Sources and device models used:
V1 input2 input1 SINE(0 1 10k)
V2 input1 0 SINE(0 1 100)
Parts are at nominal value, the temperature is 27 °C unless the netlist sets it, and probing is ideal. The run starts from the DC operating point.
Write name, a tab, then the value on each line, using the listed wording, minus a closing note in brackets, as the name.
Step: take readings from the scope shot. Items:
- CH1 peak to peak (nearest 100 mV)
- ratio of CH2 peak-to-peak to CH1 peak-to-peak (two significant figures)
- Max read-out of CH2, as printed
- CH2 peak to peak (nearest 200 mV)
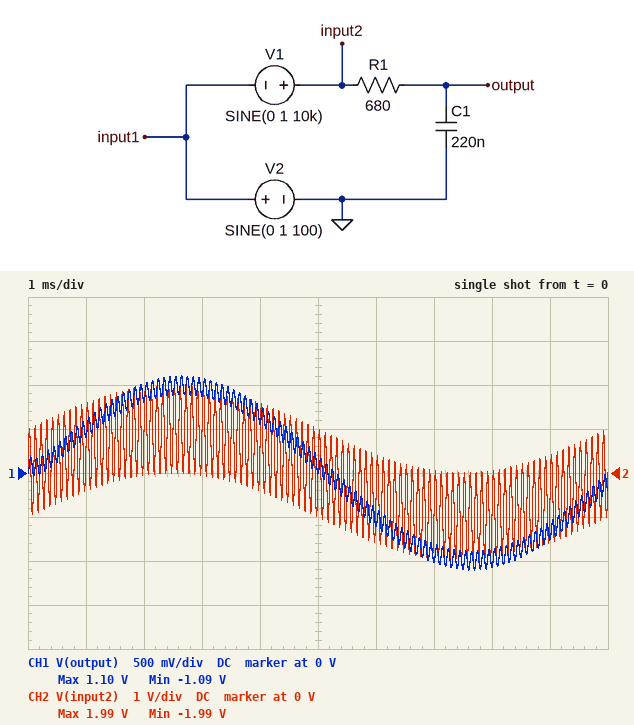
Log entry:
CH1 peak to peak	2.2 V
ratio of CH2 peak-to-peak to CH1 peak-to-peak	1.8
Max read-out of CH2, as printed	1.99 V
CH2 peak to peak	4.0 V
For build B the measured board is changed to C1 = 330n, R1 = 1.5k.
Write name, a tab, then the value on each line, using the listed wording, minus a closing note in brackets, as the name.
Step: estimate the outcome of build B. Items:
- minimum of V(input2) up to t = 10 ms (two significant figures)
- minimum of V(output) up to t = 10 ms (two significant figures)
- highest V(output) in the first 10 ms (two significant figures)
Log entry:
minimum of V(input2) up to t = 10 ms	-2.0 V
minimum of V(output) up to t = 10 ms	-990 mV
highest V(output) in the first 10 ms	990 mV
